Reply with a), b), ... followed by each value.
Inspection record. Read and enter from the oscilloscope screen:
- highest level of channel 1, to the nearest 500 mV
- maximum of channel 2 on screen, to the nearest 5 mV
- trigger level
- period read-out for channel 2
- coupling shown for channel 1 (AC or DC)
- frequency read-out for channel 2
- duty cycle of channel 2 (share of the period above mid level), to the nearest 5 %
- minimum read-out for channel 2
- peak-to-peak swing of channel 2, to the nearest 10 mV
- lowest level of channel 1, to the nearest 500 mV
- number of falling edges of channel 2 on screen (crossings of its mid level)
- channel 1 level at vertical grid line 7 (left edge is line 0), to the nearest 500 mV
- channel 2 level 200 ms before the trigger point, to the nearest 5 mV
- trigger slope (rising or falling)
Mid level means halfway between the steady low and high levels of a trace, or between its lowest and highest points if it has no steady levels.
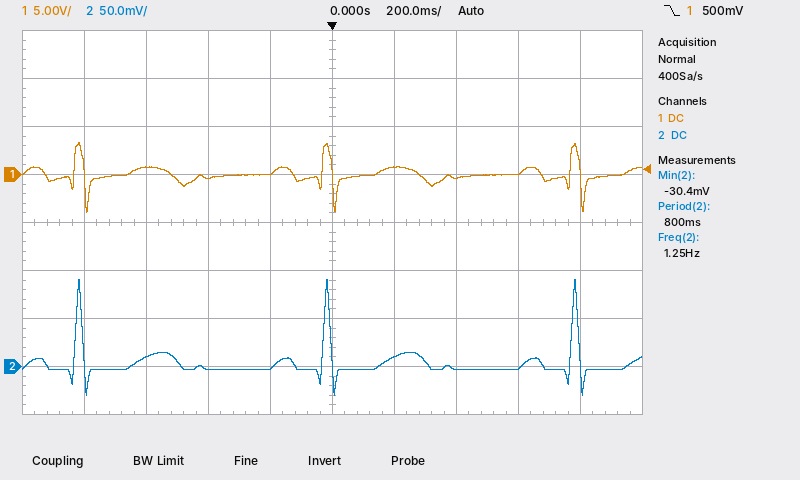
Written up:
a) 3.5 V
b) 90 mV
c) 500 mV
d) 800 ms
e) DC
f) 1.25 Hz
g) 5 %
h) -30.4 mV
i) 120 mV
j) -4.0 V
k) 3
l) -500 mV
m) 0 mV
n) falling
